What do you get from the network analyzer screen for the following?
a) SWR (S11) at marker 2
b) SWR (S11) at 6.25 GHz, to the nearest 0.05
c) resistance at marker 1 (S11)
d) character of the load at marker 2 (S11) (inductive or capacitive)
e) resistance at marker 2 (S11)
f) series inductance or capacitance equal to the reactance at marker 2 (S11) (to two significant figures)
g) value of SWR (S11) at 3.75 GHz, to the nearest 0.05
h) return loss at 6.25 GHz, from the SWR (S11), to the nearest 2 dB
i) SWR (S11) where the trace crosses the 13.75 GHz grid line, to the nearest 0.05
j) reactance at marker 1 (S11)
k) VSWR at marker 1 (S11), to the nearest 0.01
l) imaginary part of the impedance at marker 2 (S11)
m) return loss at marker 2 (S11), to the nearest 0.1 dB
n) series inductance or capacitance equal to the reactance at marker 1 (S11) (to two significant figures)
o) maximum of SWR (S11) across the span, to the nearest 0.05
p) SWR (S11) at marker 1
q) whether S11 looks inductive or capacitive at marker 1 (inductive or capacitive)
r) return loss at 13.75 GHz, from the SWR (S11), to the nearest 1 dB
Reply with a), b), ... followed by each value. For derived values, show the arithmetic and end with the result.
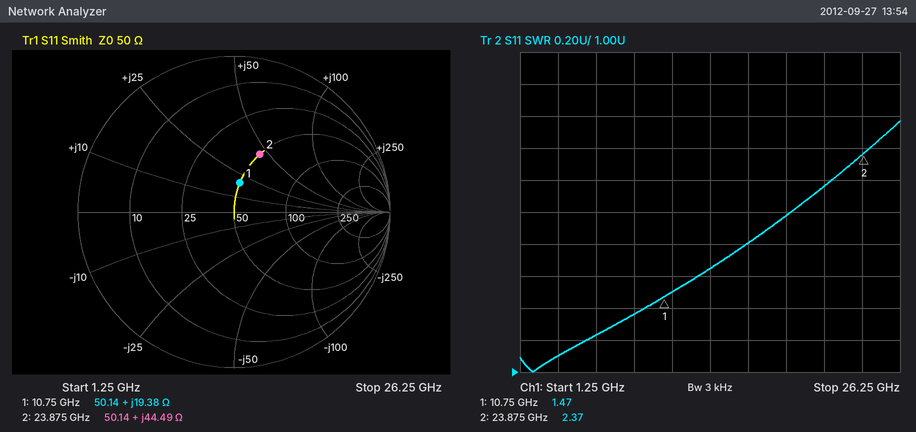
a) 2.37
b) 1.25
c) 50.14 Ω
d) inductive
e) 50.14 Ω
f) L = 44.49 Ω/(2π × 23.875 GHz) ≈ 297 pH, so 300 pH to two significant figures
g) 1.10
h) −20 log10((1.25 − 1)/(1.25 + 1)) ≈ 19.1 dB, so 20 dB to the nearest 2 dB
i) 1.65
j) +19.38 Ω
k) 1.47
l) +44.49 Ω
m) 7.8 dB
n) L = 19.38 Ω/(2π × 10.75 GHz) ≈ 287 pH, so 290 pH to two significant figures
o) 2.55
p) 1.47
q) inductive
r) −20 log10((1.65 − 1)/(1.65 + 1)) ≈ 12 dB
